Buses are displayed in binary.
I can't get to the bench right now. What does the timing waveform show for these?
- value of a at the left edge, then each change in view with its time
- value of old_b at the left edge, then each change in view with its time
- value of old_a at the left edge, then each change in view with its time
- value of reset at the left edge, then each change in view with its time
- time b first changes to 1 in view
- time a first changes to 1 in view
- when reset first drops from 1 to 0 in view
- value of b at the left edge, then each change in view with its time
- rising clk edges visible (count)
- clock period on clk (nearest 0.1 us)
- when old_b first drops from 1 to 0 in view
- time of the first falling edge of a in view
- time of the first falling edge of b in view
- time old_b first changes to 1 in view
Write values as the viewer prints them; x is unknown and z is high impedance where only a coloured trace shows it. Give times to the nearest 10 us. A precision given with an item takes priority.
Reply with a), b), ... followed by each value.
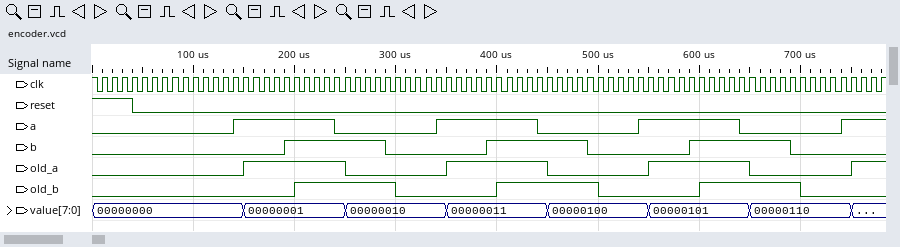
a) 0, 1 at 140 us, 0 at 240 us, 1 at 340 us, 0 at 440 us, 1 at 540 us, 0 at 640 us, 1 at 740 us
b) 0, 1 at 200 us, 0 at 300 us, 1 at 400 us, 0 at 500 us, 1 at 600 us, 0 at 700 us
c) 0, 1 at 150 us, 0 at 250 us, 1 at 350 us, 0 at 450 us, 1 at 550 us, 0 at 650 us, 1 at 750 us
d) 1, 0 at 40 us
e) 190 us
f) 140 us
g) 40 us
h) 0, 1 at 190 us, 0 at 290 us, 1 at 390 us, 0 at 490 us, 1 at 590 us, 0 at 690 us
i) 78
j) 10 us
k) 300 us
l) 240 us
m) 290 us
n) 200 us
